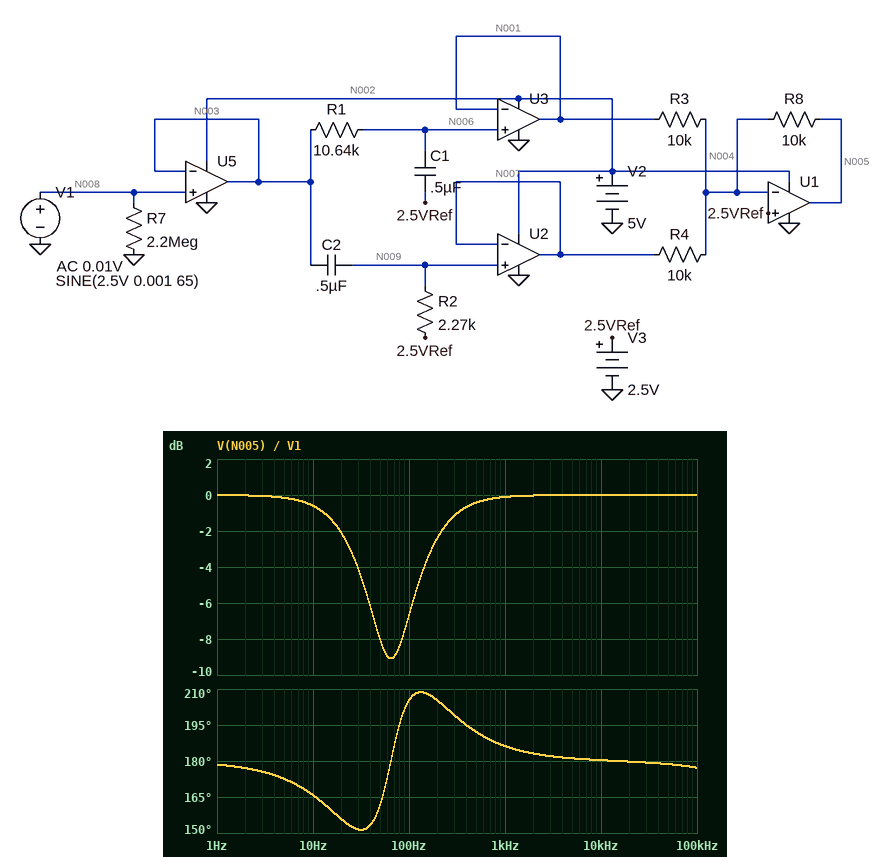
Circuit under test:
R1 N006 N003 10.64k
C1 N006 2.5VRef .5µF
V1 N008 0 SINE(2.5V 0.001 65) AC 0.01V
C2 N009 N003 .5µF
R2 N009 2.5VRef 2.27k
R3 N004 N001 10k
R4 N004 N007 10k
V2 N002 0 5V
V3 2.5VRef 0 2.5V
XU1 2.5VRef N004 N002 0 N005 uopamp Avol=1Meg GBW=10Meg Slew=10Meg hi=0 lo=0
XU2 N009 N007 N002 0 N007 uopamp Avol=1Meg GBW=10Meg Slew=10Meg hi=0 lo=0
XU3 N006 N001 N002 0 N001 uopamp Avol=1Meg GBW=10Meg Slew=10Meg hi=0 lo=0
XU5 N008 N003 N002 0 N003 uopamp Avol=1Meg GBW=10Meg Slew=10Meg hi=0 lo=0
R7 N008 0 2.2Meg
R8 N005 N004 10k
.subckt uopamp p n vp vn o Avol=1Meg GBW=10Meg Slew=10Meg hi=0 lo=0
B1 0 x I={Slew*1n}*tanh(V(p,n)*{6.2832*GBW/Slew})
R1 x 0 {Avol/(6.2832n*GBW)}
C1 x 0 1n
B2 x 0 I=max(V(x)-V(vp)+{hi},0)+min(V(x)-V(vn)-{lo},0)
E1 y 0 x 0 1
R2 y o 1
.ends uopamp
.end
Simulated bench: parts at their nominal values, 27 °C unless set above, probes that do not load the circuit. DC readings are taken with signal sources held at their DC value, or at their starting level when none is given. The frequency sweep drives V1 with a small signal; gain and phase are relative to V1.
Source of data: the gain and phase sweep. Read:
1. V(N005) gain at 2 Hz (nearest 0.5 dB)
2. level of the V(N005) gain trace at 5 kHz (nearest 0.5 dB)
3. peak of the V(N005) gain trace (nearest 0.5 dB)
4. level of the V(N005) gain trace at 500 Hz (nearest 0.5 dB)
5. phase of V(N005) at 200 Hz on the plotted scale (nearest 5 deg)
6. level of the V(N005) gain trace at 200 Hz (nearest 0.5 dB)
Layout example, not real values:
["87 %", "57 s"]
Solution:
["0 dB", "0 dB", "0 dB", "-0.5 dB", "205 deg", "-2.5 dB"]
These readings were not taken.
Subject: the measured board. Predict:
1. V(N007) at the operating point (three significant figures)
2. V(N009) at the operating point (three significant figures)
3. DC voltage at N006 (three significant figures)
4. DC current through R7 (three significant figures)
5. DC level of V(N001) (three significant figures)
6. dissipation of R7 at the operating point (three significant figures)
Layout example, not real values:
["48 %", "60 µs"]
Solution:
["2.50 V", "2.50 V", "2.50 V", "1.14 µA", "2.50 V", "2.84 µW"]
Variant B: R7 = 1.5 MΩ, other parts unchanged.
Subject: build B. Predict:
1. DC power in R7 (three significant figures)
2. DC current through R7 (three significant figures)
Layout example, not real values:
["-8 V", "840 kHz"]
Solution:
["4.17 µW", "1.67 µA"]
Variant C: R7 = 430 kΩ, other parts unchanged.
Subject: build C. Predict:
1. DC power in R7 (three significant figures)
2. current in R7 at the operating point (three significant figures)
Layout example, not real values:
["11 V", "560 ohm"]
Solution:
["14.5 µW", "5.81 µA"]
